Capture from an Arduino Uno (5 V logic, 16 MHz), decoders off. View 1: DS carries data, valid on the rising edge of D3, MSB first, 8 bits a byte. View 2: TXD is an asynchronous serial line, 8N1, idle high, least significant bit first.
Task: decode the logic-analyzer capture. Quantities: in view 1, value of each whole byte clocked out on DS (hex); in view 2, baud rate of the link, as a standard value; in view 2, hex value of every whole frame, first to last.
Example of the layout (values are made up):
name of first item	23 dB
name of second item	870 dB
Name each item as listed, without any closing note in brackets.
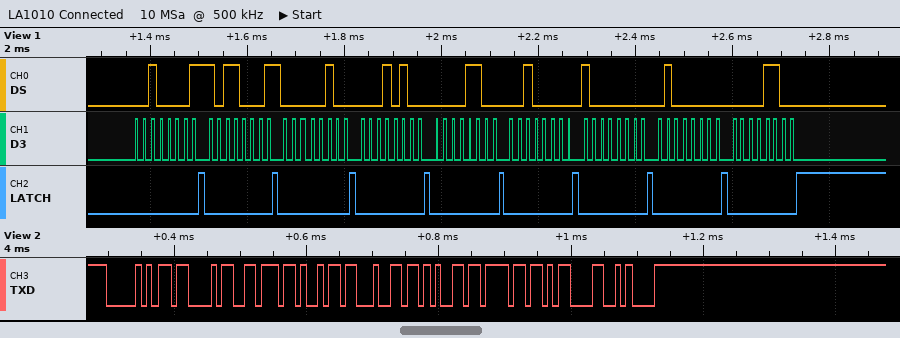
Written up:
in view 1, value of each whole byte clocked out on DS	21 B1 04 14 0C 20 80 40 0C
in view 2, baud rate of the link, as a standard value	115200 baud
in view 2, hex value of every whole frame, first to last	50 43 76 69 64 65 6F 0D 0A
